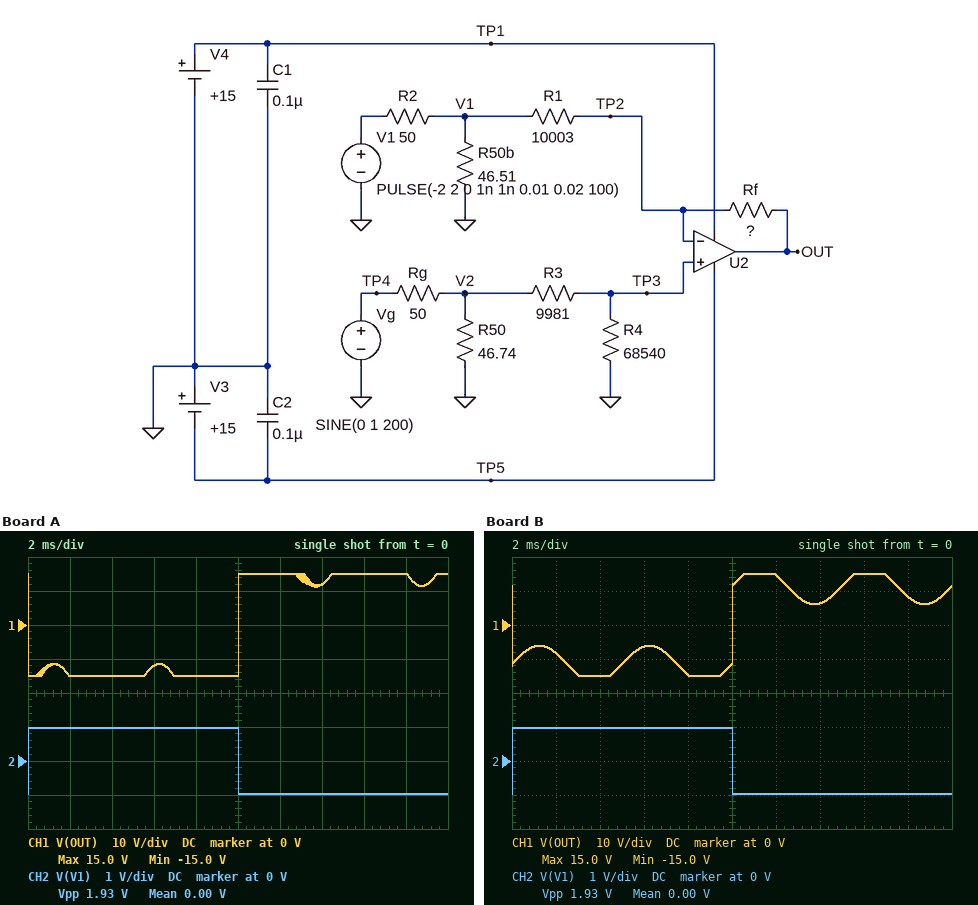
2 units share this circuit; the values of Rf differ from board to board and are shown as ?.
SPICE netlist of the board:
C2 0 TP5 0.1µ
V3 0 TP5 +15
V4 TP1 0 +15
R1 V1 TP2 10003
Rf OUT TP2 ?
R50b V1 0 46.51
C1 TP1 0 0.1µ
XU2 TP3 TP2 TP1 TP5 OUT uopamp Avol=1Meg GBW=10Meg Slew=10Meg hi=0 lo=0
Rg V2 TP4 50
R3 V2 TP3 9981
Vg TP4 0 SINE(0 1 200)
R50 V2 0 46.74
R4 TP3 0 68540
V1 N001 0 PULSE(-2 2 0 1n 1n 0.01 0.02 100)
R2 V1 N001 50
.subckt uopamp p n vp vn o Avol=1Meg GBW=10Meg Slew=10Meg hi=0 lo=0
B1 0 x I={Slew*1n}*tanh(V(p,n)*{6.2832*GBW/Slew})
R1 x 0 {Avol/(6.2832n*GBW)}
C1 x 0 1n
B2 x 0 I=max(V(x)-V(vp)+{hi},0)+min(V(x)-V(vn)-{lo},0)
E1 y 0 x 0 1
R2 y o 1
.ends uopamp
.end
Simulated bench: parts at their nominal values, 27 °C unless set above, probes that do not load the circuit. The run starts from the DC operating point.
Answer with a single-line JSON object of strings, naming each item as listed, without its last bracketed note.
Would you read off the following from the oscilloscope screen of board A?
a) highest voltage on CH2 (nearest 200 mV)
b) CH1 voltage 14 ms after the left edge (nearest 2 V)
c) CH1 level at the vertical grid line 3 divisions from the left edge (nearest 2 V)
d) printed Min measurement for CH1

{"highest voltage on CH2": "1.0 V", "CH1 voltage 14 ms after the left edge": "12 V", "CH1 level at the vertical grid line 3 divisions from the left edge": "-12 V", "printed Min measurement for CH1": "-15.0 V"}
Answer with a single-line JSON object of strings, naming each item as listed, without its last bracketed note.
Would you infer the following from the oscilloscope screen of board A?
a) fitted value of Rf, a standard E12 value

{"fitted value of Rf, a standard E12 value": "220 kΩ"}
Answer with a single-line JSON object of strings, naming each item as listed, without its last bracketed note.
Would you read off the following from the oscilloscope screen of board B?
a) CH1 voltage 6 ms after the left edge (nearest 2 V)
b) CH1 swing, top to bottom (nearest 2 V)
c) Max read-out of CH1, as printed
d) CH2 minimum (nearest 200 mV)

{"CH1 voltage 6 ms after the left edge": "-6 V", "CH1 swing, top to bottom": "30 V", "Max read-out of CH1, as printed": "15.0 V", "CH2 minimum": "-1.0 V"}
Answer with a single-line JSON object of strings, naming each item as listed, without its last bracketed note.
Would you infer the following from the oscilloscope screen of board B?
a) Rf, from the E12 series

{"Rf, from the E12 series": "120 kΩ"}
